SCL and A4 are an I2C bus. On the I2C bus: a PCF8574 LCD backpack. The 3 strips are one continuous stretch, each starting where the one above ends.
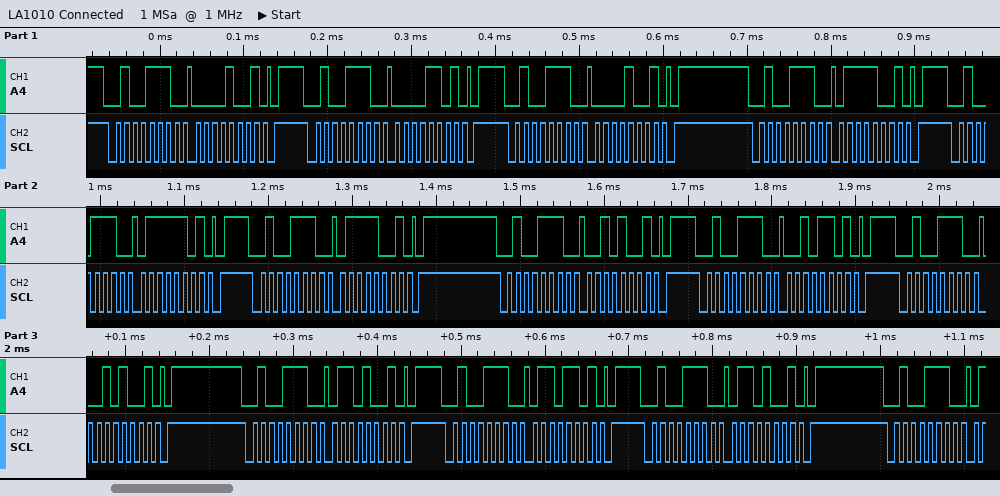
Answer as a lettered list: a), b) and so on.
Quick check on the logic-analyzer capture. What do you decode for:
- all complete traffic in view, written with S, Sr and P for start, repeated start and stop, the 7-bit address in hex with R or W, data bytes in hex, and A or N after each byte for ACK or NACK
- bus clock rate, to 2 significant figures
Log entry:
a) S 27W A 09 A P S 27W A 0D A P S 27W A 09 A P S 27W A 79 A P S 27W A 7D A P S 27W A 79 A P S 27W A 29 A P S 27W A 2D A P S 27W A 29 A P S 27W A 69 A P S 27W A 6D A P S 27W A 69 A P S 27W A
b) 100 kHz
